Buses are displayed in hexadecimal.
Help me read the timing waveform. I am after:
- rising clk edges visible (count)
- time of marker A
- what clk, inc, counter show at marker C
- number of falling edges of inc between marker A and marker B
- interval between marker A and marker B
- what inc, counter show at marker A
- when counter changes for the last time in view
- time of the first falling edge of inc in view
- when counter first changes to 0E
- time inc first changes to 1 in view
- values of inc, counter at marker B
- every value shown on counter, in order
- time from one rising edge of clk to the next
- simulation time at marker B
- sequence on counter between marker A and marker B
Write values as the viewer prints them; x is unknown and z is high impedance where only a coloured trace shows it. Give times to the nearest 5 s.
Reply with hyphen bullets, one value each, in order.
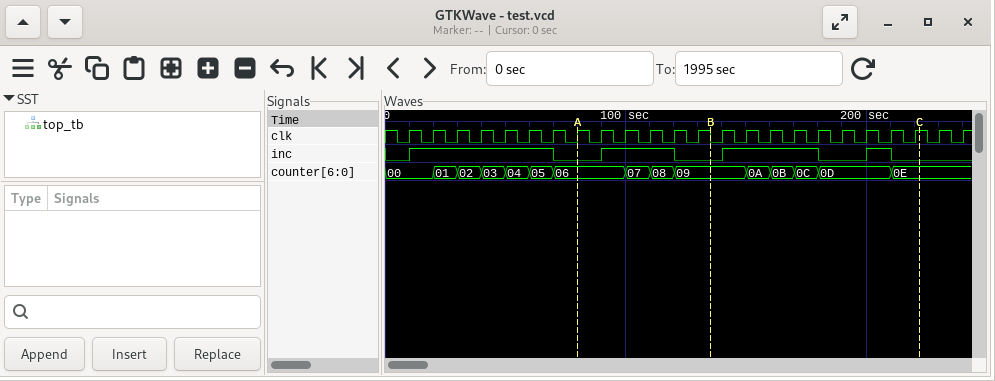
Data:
- 24
- 80 s
- clk=1, inc=0, counter=0E
- 1
- 55 s
- inc=0, counter=06
- 210 s
- 70 s
- 210 s
- 10 s
- inc=0, counter=09
- 00, 01, 02, 03, 04, 05, 06, 07, 08, 09, 0A, 0B, 0C, 0D, 0E
- 10 s
- 135 s
- 06, 07, 08, 09
